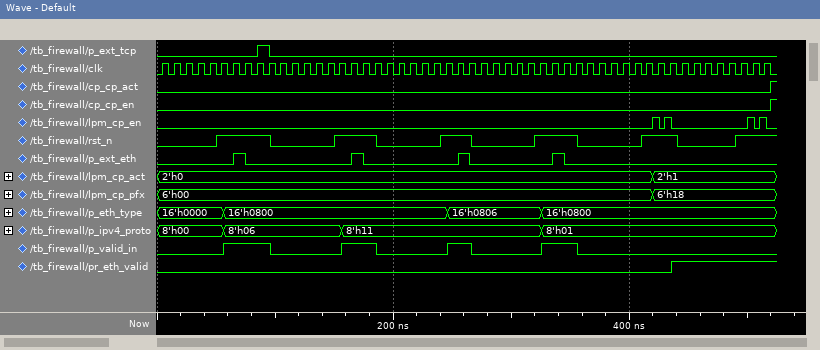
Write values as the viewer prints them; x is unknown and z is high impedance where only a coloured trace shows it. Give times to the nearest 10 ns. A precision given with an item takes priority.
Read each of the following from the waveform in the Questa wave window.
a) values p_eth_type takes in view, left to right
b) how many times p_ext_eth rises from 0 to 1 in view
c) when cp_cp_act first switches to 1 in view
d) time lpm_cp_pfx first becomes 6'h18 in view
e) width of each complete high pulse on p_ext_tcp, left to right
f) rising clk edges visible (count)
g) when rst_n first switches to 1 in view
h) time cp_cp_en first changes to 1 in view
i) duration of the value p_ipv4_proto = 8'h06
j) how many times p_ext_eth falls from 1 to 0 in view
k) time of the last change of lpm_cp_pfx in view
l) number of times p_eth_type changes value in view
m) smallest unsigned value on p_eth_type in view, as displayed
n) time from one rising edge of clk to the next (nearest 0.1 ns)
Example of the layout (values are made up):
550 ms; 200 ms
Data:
16'h0000, 16'h0800, 16'h0806, 16'h0800; 4; 520 ns; 420 ns; 10 ns; 52; 50 ns; 520 ns; 100 ns; 4; 420 ns; 3; 16'h0000; 10 ns
